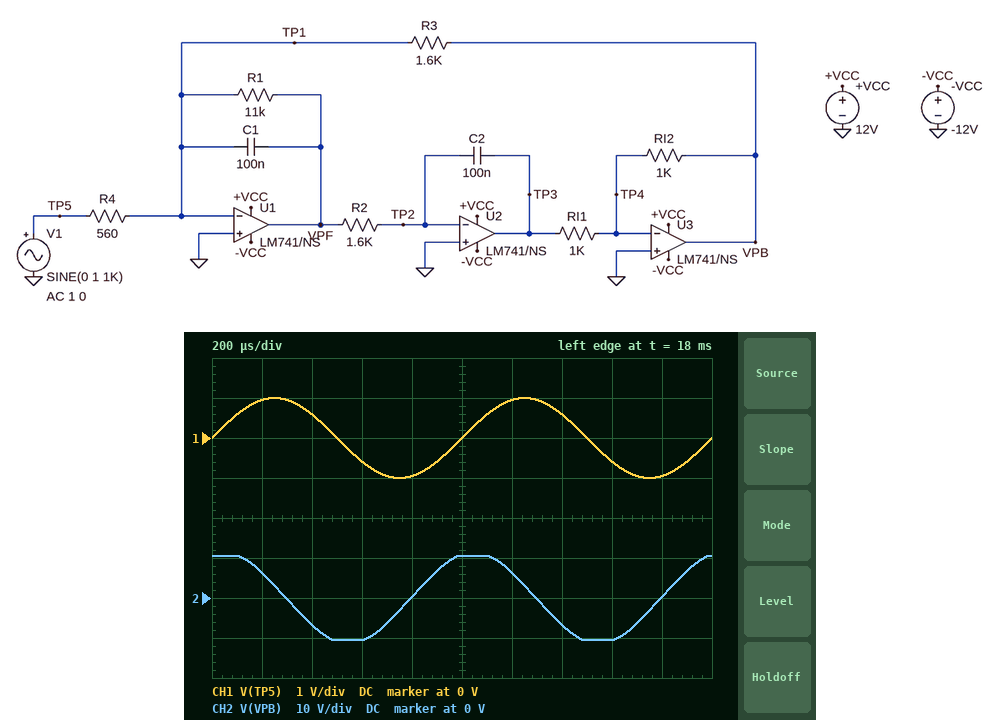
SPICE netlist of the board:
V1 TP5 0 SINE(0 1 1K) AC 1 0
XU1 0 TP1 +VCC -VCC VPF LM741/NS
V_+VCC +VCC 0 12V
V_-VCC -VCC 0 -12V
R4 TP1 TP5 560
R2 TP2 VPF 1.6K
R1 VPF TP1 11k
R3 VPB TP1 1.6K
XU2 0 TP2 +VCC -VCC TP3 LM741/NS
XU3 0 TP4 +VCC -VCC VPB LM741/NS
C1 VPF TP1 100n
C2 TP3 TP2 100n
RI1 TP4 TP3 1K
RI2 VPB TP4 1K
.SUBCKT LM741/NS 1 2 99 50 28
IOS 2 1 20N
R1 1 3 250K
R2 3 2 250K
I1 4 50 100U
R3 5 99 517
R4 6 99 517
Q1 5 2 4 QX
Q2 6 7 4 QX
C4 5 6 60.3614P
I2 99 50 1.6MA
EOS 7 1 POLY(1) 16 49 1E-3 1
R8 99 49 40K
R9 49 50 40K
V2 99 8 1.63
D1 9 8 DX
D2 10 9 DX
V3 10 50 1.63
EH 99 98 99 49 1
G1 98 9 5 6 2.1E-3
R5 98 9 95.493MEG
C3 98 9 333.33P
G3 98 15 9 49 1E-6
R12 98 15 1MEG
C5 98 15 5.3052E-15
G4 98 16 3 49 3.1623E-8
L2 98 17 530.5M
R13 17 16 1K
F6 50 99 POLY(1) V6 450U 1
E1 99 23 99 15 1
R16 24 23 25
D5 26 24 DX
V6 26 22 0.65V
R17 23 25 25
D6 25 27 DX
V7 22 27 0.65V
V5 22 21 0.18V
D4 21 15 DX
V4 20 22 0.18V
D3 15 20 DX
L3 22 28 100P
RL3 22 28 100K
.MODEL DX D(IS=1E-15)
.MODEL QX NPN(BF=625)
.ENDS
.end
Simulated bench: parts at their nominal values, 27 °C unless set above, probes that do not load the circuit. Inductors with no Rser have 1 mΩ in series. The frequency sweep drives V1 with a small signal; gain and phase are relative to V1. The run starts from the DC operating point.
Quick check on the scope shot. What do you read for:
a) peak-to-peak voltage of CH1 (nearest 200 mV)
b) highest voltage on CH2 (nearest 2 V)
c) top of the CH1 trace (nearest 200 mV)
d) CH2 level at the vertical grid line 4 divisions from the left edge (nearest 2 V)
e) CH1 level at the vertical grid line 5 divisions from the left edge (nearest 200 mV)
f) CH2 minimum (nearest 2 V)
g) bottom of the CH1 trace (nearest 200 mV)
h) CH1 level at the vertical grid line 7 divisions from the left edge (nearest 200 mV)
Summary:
2.0 V
10 V
1.0 V
0 V
0 V
-10 V
-1.0 V
600 mV
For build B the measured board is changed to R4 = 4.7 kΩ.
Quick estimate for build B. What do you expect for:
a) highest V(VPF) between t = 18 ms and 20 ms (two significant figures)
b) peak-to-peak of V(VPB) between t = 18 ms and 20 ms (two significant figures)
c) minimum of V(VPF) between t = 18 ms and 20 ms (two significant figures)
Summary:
2.4 V
4.8 V
-2.4 V
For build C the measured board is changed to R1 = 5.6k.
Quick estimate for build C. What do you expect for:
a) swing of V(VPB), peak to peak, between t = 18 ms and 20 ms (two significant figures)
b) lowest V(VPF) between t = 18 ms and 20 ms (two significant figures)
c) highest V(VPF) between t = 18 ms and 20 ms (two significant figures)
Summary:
20 V
-10 V
10 V
